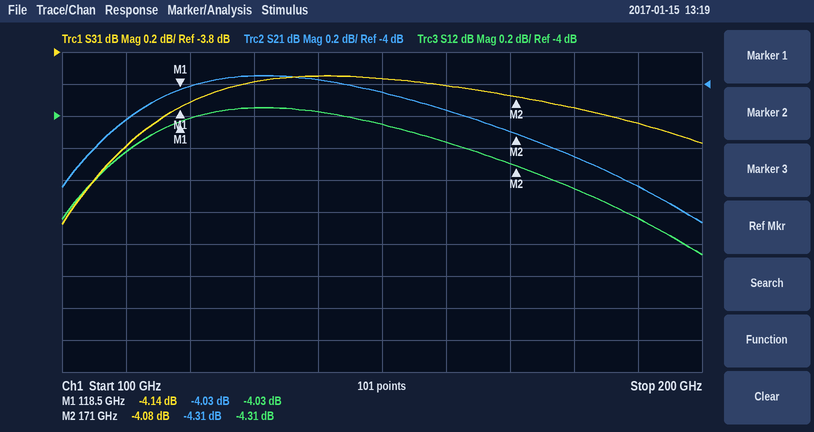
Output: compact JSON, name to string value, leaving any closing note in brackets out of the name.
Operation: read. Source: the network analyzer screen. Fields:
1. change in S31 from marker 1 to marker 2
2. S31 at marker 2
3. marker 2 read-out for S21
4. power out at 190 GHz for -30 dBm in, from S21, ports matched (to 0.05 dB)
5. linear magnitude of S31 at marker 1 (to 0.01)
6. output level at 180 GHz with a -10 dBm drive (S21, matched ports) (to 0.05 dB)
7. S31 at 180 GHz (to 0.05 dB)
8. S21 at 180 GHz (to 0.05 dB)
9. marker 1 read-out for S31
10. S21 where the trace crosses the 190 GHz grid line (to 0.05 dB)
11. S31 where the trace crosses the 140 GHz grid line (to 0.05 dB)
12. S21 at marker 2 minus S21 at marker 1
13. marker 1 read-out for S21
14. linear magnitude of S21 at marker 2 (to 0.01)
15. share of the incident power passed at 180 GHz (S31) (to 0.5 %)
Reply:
{"change in S31 from marker 1 to marker 2": "0.06 dB", "S31 at marker 2": "-4.08 dB", "marker 2 read-out for S21": "-4.31 dB", "power out at 190 GHz for -30 dBm in, from S21, ports matched": "-34.65 dBm", "linear magnitude of S31 at marker 1": "0.62", "output level at 180 GHz with a -10 dBm drive (S21, matched ports)": "-14.45 dBm", "S31 at 180 GHz": "-4.15 dB", "S21 at 180 GHz": "-4.45 dB", "marker 1 read-out for S31": "-4.14 dB", "S21 where the trace crosses the 190 GHz grid line": "-4.65 dB", "S31 where the trace crosses the 140 GHz grid line": "-3.95 dB", "S21 at marker 2 minus S21 at marker 1": "-0.28 dB", "marker 1 read-out for S21": "-4.03 dB", "linear magnitude of S21 at marker 2": "0.61", "share of the incident power passed at 180 GHz (S31)": "38.5 %"}
